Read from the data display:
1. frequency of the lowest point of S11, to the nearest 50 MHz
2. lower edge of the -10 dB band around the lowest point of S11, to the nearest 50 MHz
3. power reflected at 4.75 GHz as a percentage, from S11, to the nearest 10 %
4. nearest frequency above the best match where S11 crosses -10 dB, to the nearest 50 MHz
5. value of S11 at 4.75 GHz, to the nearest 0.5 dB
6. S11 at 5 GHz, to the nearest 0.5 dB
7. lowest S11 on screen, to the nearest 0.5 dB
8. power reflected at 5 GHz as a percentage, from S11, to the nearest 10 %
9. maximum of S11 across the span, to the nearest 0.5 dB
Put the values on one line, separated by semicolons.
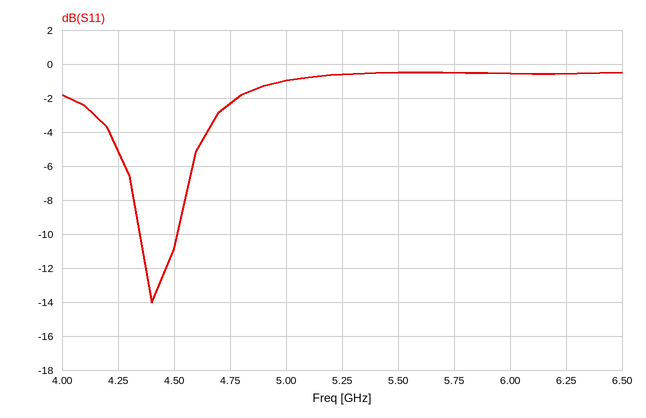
4.40 GHz; 4.35 GHz; 60 %; 4.50 GHz; -2.5 dB; -1.0 dB; -14.0 dB; 80 %; -0.5 dB
